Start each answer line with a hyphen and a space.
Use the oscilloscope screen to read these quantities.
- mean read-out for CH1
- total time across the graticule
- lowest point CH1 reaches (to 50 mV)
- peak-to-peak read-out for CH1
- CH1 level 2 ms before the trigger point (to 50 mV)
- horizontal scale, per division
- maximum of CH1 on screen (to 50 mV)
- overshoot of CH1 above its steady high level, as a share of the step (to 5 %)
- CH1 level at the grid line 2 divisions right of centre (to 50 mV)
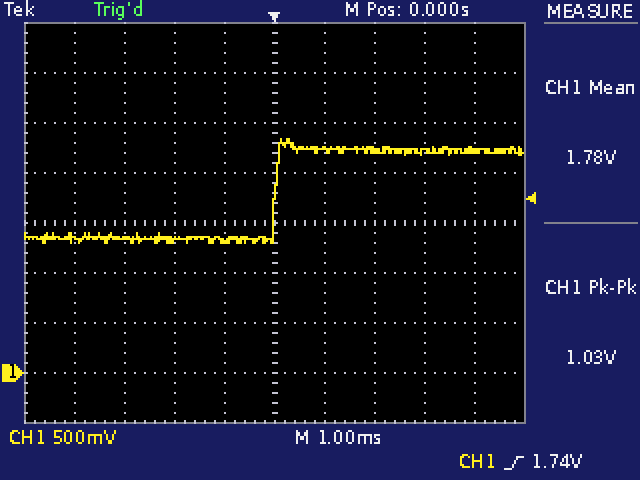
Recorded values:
- 1.78 V
- 10 ms
- 1.30 V
- 1.03 V
- 1.35 V
- 1 ms
- 2.35 V
- 10 %
- 2.25 V
